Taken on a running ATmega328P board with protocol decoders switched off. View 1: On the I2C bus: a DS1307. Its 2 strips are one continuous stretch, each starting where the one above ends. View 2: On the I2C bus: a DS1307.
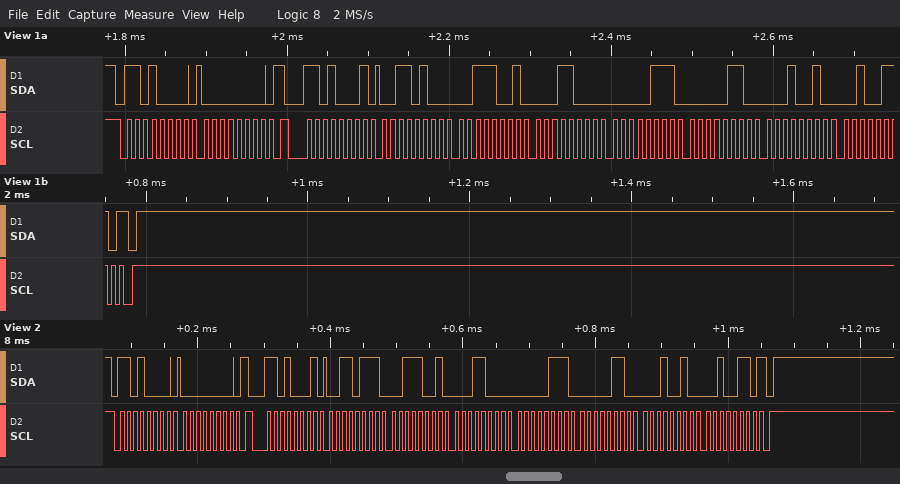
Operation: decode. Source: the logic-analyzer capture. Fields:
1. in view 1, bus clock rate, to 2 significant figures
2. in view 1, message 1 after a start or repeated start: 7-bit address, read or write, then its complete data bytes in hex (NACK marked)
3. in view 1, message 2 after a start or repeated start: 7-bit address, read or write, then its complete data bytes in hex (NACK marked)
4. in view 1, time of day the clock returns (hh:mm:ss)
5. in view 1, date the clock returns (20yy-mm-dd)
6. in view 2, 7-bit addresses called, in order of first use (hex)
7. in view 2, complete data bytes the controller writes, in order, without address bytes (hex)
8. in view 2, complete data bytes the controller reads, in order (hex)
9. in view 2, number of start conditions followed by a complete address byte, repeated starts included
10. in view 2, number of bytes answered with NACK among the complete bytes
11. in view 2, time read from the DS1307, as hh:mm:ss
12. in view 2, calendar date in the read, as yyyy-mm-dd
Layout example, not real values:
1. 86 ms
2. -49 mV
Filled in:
1. 100 kHz
2. 0x68 write: 00
3. 0x68 read: 34 39 18 07 06 12 26 NACK
4. 18:39:34
5. 2026-12-06
6. 0x68
7. 00
8. 37 39 18 07 06 12 26
9. 2
10. 1
11. 18:39:37
12. 2026-12-06
